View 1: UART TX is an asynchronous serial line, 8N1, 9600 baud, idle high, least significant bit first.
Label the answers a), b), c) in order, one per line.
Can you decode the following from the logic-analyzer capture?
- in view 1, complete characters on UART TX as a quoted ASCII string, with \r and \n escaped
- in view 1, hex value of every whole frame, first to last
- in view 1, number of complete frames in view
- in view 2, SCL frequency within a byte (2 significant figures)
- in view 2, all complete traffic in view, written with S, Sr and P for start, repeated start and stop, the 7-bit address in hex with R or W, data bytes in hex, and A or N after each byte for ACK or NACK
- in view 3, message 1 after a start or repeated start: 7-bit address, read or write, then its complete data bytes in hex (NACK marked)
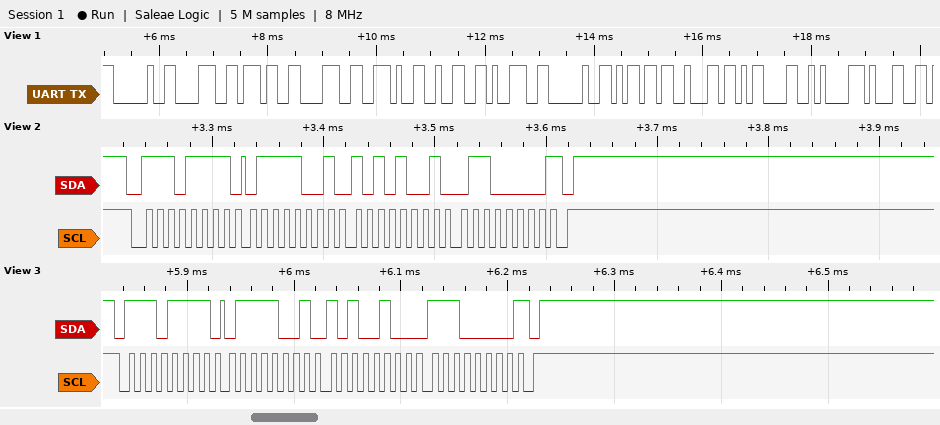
a) " 878.29 mb\r\n1"
b) 20 38 37 38 2E 32 39 20 6D 62 0D 0A 31
c) 13
d) 100 kHz
e) S 77R A 79 A A9 A 60 N P
f) 0x77 read: 79 A4 E0 NACK
